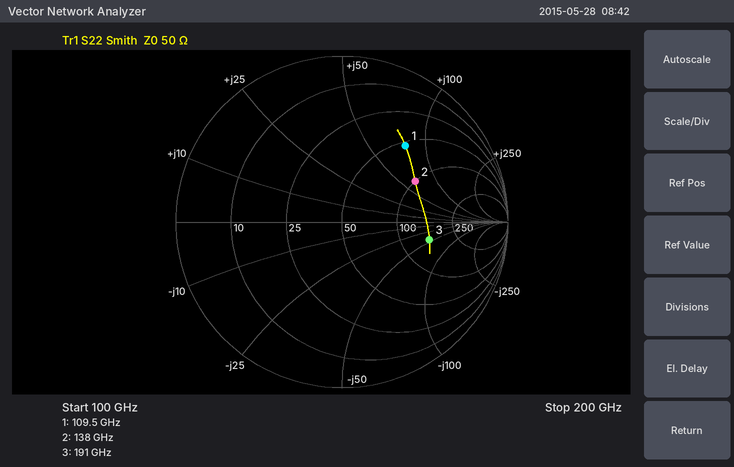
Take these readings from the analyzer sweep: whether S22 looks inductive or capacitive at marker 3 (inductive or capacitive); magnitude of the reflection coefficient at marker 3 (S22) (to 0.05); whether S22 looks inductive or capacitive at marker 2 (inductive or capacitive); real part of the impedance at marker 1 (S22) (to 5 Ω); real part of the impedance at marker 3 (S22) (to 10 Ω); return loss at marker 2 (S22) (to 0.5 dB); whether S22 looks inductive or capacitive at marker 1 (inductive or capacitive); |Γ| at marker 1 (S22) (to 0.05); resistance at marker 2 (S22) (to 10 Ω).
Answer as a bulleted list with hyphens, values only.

- capacitive
- 0.55
- inductive
- 55 Ω
- 150 Ω
- 6.0 dB
- inductive
- 0.60
- 100 Ω
